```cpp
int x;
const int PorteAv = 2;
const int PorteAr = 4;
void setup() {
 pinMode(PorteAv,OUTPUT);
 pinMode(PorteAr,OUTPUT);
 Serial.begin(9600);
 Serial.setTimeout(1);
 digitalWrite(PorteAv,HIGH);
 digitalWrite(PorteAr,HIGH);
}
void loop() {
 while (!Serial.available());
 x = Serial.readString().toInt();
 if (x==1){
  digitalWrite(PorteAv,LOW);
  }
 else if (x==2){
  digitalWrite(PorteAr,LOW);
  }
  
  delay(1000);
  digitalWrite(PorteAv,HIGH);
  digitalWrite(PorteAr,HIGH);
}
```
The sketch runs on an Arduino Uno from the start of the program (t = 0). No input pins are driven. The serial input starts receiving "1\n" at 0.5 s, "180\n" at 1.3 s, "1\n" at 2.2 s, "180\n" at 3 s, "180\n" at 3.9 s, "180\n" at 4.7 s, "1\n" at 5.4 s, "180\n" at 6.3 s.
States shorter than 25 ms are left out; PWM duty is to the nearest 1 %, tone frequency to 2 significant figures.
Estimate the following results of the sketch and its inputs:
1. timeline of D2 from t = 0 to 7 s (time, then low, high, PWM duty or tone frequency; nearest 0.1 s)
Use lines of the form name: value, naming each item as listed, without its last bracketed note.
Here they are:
timeline of D2 from t = 0 to 7 s: 0 s high; 0.5 s low; 1.5 s high; 2.5 s low; 3.5 s high
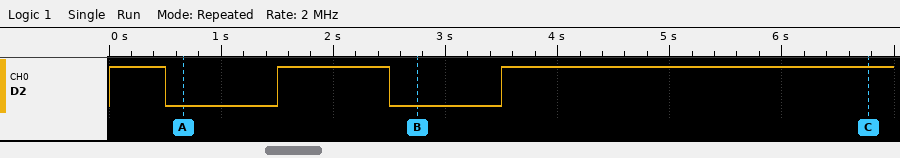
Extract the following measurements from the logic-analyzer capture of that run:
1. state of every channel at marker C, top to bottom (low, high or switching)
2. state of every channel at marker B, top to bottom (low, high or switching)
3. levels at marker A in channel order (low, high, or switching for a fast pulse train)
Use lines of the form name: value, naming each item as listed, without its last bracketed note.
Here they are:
state of every channel at marker C, top to bottom: D2 high
state of every channel at marker B, top to bottom: D2 low
levels at marker A in channel order: D2 low
